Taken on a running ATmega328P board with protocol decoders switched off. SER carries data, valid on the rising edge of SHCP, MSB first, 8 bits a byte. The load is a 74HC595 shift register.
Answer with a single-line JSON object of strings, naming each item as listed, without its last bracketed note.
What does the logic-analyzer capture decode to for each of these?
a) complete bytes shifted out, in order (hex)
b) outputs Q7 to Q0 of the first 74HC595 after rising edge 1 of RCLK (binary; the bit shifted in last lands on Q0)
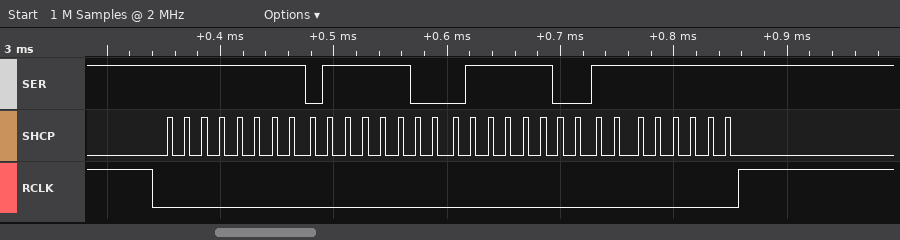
{"complete bytes shifted out, in order": "FF 7C 7C FF", "outputs Q7 to Q0 of the first 74HC595 after rising edge 1 of RCLK": "11111111"}
